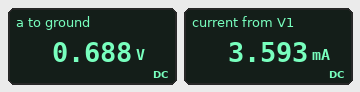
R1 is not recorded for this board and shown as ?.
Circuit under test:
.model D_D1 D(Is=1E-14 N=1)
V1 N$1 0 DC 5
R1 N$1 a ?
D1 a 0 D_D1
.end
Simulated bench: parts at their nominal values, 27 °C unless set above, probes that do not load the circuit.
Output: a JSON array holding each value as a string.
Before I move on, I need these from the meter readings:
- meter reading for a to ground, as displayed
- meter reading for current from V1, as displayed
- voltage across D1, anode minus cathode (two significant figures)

["0.688 V", "3.593 mA", "690 mV"]
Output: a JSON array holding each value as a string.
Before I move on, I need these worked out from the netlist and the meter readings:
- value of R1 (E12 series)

["1.2 kΩ"]
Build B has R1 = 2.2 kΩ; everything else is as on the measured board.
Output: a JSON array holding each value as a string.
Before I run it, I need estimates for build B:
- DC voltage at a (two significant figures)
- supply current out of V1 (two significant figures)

["670 mV", "2.0 mA"]
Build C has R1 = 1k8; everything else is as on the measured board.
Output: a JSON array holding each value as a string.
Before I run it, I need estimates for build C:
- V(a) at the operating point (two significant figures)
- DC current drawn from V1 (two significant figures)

["680 mV", "2.4 mA"]
